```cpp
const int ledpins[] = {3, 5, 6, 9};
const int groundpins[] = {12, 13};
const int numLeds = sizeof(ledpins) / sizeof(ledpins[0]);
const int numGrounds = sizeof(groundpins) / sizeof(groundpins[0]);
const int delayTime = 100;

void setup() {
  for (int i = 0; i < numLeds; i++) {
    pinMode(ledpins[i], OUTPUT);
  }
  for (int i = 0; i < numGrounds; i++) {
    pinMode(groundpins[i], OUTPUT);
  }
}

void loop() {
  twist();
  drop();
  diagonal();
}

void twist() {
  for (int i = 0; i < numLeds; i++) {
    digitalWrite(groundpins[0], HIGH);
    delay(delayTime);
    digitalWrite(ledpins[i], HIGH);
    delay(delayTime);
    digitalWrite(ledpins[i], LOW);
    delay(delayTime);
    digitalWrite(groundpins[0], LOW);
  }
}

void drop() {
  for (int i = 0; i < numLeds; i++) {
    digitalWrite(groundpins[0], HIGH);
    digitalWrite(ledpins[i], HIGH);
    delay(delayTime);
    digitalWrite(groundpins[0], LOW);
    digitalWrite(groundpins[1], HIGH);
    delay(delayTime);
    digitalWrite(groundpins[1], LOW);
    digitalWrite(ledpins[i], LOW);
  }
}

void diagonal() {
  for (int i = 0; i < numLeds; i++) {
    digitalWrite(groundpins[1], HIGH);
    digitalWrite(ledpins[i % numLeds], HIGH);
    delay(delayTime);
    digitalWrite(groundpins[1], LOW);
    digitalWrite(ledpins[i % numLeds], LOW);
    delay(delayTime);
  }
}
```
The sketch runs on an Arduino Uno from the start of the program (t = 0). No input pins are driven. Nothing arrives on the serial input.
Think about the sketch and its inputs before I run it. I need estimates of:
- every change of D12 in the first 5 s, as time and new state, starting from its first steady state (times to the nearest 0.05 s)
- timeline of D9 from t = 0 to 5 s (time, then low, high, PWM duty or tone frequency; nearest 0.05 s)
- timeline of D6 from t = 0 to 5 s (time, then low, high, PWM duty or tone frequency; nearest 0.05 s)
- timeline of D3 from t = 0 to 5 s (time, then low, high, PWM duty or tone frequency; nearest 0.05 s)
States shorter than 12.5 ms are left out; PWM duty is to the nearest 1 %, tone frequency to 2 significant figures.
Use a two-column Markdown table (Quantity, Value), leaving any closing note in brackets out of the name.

| Quantity | Value |
|---|---|
| every change of D12 in the first 5 s, as time and new state, starting from its first steady state | 0 s high; 1.3 s low; 1.4 s high; 1.5 s low; 1.6 s high; 1.7 s low; 1.8 s high; 1.9 s low; 2.8 s high; 4.1 s low; 4.2 s high; 4.3 s low; 4.4 s high; 4.5 s low; 4.6 s high; 4.7 s low |
| timeline of D9 from t = 0 to 5 s | 0 s low; 1 s high; 1.1 s low; 1.8 s high; 2 s low; 2.6 s high; 2.7 s low; 3.8 s high; 3.9 s low; 4.6 s high; 4.8 s low |
| timeline of D6 from t = 0 to 5 s | 0 s low; 0.7 s high; 0.8 s low; 1.6 s high; 1.8 s low; 2.4 s high; 2.5 s low; 3.5 s high; 3.6 s low; 4.4 s high; 4.6 s low |
| timeline of D3 from t = 0 to 5 s | 0 s low; 0.1 s high; 0.2 s low; 1.2 s high; 1.4 s low; 2 s high; 2.1 s low; 2.9 s high; 3 s low; 4 s high; 4.2 s low; 4.8 s high; 4.9 s low |
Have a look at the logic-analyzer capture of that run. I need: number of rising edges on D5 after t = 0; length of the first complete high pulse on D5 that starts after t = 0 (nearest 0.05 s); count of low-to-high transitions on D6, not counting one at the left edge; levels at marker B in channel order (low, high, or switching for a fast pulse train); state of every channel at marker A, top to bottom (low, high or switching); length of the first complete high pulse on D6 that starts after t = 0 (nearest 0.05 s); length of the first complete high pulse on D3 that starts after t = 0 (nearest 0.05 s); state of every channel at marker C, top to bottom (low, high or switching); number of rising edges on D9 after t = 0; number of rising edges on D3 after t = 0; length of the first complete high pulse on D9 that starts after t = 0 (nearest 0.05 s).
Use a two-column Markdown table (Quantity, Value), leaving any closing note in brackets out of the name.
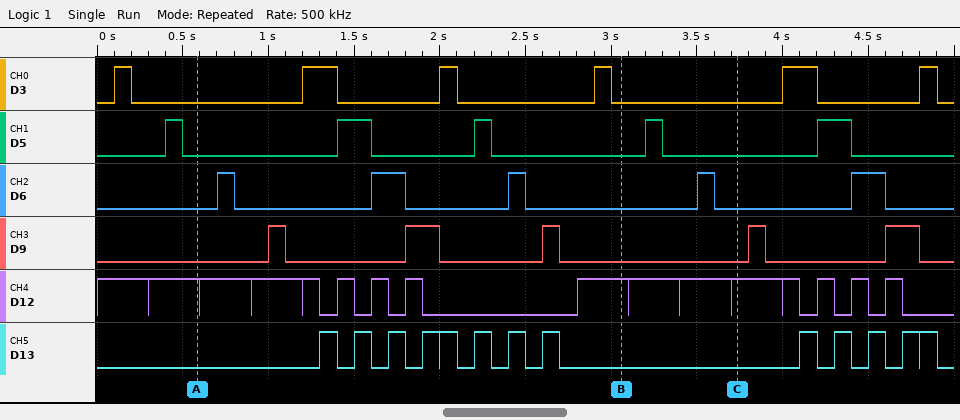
| Quantity | Value |
|---|---|
| number of rising edges on D5 after t = 0 | 5 |
| length of the first complete high pulse on D5 that starts after t = 0 | 0.10 s |
| count of low-to-high transitions on D6, not counting one at the left edge | 5 |
| levels at marker B in channel order | D3 low, D5 low, D6 low, D9 low, D12 high, D13 low |
| state of every channel at marker A, top to bottom | D3 low, D5 low, D6 low, D9 low, D12 high, D13 low |
| length of the first complete high pulse on D6 that starts after t = 0 | 0.10 s |
| length of the first complete high pulse on D3 that starts after t = 0 | 0.10 s |
| state of every channel at marker C, top to bottom | D3 low, D5 low, D6 low, D9 low, D12 high, D13 low |
| number of rising edges on D9 after t = 0 | 5 |
| number of rising edges on D3 after t = 0 | 6 |
| length of the first complete high pulse on D9 that starts after t = 0 | 0.10 s |
